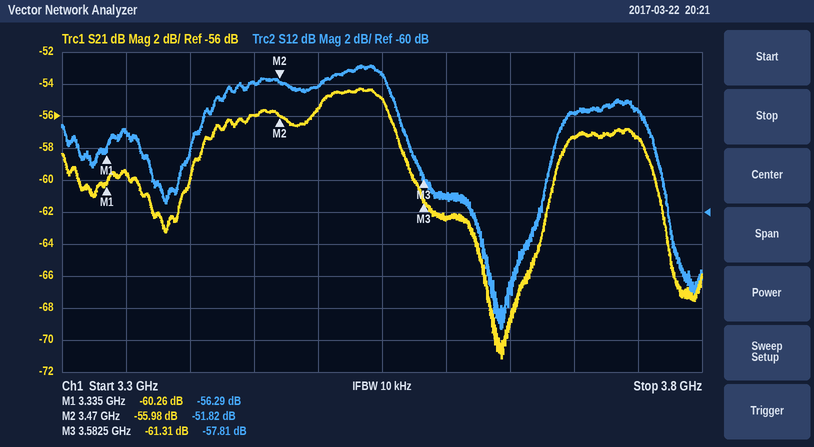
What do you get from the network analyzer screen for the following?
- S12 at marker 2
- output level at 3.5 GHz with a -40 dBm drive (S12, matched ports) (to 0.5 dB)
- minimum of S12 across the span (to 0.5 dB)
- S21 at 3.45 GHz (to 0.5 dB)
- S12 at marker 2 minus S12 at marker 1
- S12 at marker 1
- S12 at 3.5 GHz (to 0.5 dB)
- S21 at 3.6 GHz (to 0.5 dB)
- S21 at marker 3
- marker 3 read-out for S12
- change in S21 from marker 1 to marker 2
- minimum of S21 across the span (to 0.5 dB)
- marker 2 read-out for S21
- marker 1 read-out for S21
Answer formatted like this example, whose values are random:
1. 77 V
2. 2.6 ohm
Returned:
1. -51.82 dB
2. -92.0 dBm
3. -67.5 dB
4. -56.0 dB
5. 4.47 dB
6. -56.29 dB
7. -52.0 dB
8. -62.5 dB
9. -61.31 dB
10. -57.81 dB
11. 4.28 dB
12. -71.0 dB
13. -55.98 dB
14. -60.26 dB
